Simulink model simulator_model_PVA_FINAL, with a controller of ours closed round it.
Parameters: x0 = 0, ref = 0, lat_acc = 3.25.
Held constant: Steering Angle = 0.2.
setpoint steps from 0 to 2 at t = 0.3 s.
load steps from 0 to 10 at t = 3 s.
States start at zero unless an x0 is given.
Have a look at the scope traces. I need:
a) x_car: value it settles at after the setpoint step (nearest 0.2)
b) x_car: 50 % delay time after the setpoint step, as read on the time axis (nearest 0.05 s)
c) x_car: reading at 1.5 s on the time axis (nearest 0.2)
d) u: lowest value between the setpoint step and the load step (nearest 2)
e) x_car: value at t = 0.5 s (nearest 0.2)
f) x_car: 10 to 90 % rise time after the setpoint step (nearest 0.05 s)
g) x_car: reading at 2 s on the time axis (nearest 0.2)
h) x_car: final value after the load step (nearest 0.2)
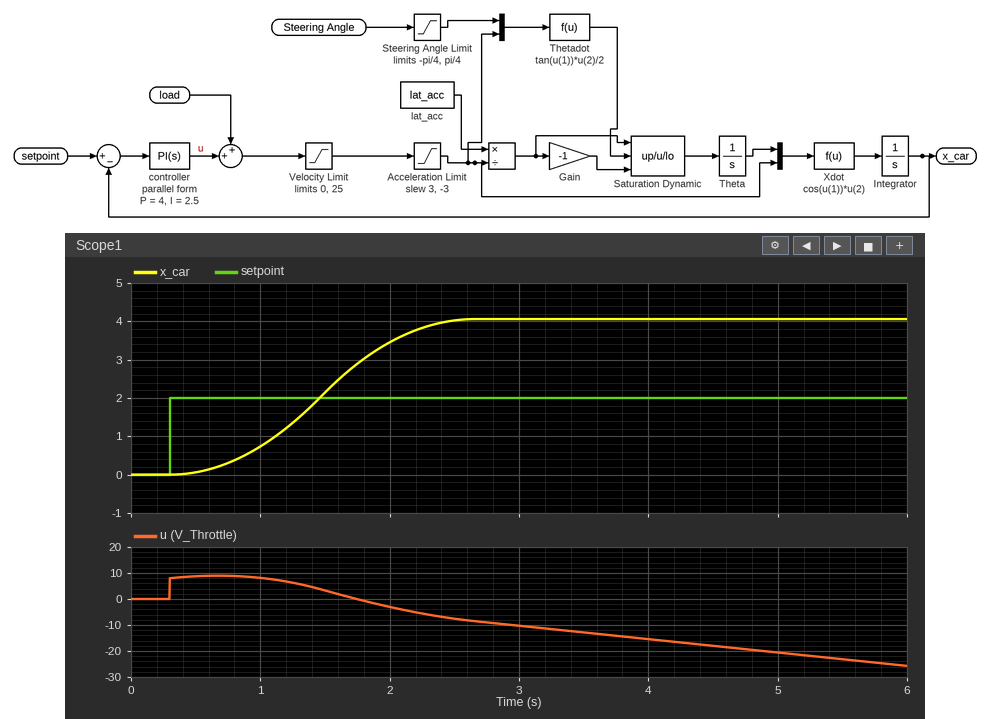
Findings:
4.0
1.45 s
2.2
-10
0.0
1.30 s
3.4
4.0
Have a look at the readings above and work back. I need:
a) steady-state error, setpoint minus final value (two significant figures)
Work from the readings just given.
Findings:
-2.0
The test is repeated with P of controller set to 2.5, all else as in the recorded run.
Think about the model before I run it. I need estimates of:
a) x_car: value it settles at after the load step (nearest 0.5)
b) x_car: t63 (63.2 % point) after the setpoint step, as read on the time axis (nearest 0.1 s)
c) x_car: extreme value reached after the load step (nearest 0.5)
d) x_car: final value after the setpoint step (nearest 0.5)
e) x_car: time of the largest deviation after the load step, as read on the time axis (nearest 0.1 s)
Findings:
4.5
1.6 s
4.5
4.0
3.5 s
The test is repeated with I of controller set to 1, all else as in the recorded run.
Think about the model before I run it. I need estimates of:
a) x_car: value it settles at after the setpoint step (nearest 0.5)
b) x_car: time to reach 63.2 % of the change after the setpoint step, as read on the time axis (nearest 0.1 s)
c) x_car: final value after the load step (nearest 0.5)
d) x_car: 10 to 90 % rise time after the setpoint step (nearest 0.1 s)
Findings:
3.0
1.5 s
4.5
1.1 s
